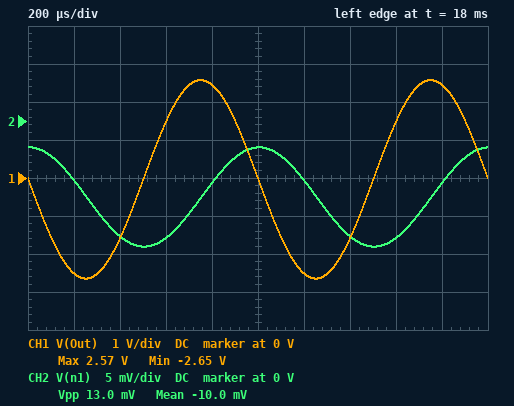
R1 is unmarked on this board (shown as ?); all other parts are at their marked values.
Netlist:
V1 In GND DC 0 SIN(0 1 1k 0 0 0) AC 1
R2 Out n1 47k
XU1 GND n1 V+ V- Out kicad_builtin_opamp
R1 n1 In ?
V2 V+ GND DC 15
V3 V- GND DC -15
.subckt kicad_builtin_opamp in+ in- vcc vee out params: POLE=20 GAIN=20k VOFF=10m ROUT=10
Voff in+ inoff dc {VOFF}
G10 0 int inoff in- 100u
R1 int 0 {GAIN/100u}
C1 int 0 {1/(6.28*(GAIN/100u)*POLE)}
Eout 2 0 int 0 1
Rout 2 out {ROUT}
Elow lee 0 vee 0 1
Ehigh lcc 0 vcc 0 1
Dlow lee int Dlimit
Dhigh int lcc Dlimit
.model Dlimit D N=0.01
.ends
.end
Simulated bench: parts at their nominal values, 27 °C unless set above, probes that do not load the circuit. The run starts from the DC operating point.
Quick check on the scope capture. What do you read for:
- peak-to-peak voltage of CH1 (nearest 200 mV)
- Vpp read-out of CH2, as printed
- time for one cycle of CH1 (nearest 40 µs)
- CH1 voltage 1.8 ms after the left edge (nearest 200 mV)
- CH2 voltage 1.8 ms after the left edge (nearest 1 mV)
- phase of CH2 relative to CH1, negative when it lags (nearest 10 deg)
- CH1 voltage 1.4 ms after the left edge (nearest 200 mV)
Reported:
5.2 V
13.0 mV
1.00 ms
2.4 V
-8 mV
-90 deg
-1.6 V
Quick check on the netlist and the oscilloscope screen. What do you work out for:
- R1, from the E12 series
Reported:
18 kΩ
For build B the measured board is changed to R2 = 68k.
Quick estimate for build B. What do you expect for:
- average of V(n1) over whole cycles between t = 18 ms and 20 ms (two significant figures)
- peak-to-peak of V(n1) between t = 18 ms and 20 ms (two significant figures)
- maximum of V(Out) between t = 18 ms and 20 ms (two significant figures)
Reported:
-10 mV
19 mV
3.7 V
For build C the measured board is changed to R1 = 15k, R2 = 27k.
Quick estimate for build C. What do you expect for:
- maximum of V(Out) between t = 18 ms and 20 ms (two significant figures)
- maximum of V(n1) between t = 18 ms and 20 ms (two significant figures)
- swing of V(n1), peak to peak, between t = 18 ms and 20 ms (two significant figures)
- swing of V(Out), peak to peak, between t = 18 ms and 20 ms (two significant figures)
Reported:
1.8 V
-5.5 mV
9.0 mV
3.6 V
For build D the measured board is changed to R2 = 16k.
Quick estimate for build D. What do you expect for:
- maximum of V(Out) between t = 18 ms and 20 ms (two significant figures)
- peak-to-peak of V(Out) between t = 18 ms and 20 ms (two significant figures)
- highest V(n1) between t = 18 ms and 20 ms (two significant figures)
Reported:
870 mV
1.8 V
-7.8 mV
